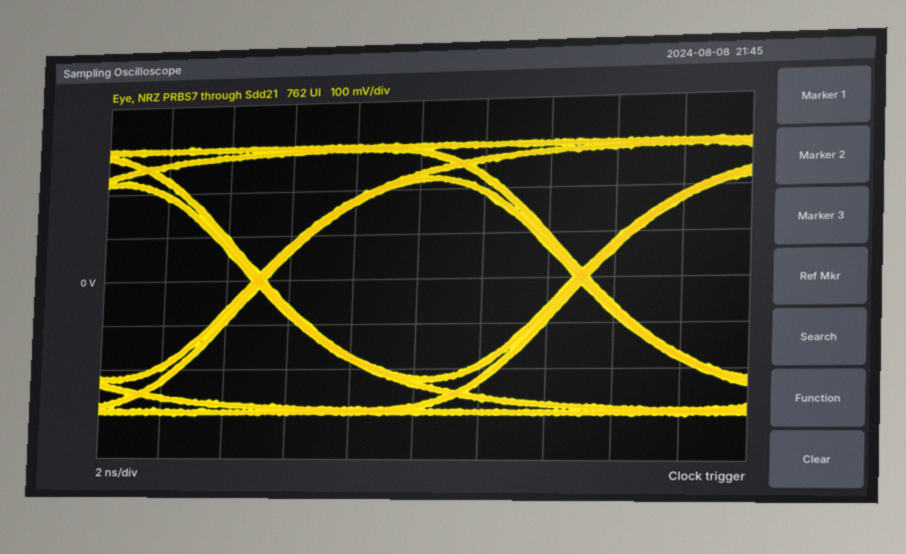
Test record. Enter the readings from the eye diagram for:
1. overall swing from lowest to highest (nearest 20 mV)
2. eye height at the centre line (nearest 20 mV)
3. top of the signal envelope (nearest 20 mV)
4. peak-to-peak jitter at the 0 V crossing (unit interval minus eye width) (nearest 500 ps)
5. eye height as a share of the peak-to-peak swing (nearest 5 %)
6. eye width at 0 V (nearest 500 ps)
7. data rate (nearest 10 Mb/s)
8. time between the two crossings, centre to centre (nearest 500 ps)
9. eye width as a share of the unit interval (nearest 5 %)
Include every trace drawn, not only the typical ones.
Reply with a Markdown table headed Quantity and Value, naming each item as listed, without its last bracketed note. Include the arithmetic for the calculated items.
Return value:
| Quantity | Value |
|---|---|
| overall swing from lowest to highest | 620 mV |
| eye height at the centre line | 440 mV |
| top of the signal envelope | 300 mV |
| peak-to-peak jitter at the 0 V crossing (unit interval minus eye width) | 500 ps |
| eye height as a share of the peak-to-peak swing | 440 mV / 620 mV ≈ 71.0 %, so 70 % to the nearest 5 % |
| eye width at 0 V | 9.5 ns |
| data rate | 100 Mb/s |
| time between the two crossings, centre to centre | 10.0 ns |
| eye width as a share of the unit interval | 9.5 ns / 10.0 ns ≈ 95 % |
